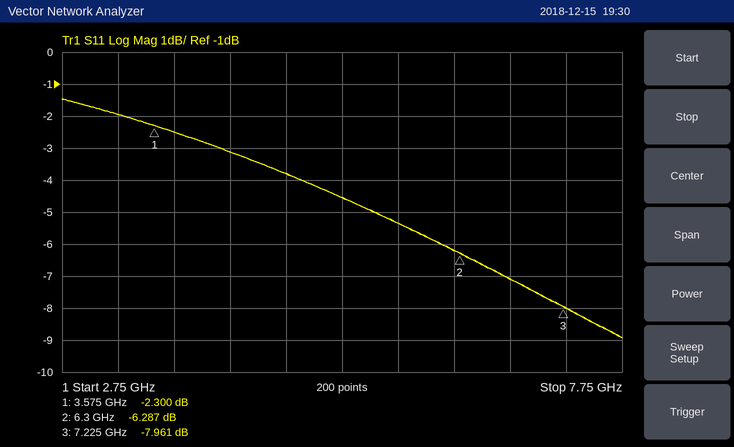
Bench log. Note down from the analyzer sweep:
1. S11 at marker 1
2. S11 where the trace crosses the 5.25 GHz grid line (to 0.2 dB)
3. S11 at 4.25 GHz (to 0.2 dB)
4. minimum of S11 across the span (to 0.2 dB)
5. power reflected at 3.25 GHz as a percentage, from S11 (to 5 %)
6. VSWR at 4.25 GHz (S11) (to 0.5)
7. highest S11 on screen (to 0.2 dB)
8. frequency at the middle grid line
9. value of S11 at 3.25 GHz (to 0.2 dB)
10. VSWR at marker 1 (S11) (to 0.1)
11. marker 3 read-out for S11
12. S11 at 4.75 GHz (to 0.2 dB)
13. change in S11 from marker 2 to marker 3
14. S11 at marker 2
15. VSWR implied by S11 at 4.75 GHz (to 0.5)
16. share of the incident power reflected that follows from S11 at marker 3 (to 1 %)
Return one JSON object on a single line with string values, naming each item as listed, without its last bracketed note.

{"S11 at marker 1": "-2.300 dB", "S11 where the trace crosses the 5.25 GHz grid line": "-4.6 dB", "S11 at 4.25 GHz": "-3.2 dB", "minimum of S11 across the span": "-9.0 dB", "power reflected at 3.25 GHz as a percentage, from S11": "65 %", "VSWR at 4.25 GHz (S11)": "5.5", "highest S11 on screen": "-1.4 dB", "frequency at the middle grid line": "5.25 GHz", "value of S11 at 3.25 GHz": "-2.0 dB", "VSWR at marker 1 (S11)": "7.6", "marker 3 read-out for S11": "-7.961 dB", "S11 at 4.75 GHz": "-3.8 dB", "change in S11 from marker 2 to marker 3": "-1.674 dB", "S11 at marker 2": "-6.287 dB", "VSWR implied by S11 at 4.75 GHz": "4.5", "share of the incident power reflected that follows from S11 at marker 3": "16 %"}
